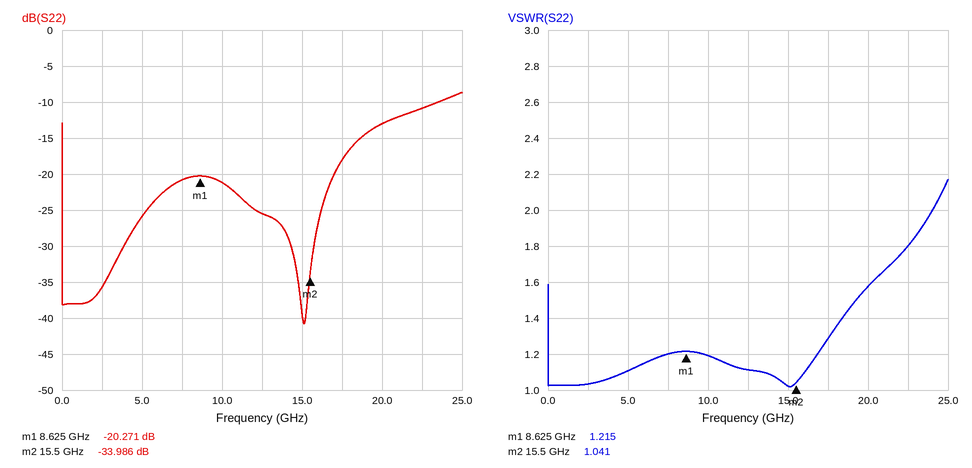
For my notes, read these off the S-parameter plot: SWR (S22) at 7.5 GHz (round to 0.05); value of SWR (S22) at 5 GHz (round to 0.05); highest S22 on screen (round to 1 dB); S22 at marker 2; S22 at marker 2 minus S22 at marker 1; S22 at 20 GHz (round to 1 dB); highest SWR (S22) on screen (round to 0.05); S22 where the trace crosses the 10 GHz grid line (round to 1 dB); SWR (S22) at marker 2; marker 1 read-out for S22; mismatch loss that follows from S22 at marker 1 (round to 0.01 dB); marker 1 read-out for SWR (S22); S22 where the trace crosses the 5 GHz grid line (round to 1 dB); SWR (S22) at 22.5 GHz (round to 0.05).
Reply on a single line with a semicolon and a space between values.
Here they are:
1.20; 1.10; -9 dB; -33.986 dB; -13.715 dB; -13 dB; 2.15; -21 dB; 1.041; -20.271 dB; 0.04 dB; 1.215; -26 dB; 1.80
